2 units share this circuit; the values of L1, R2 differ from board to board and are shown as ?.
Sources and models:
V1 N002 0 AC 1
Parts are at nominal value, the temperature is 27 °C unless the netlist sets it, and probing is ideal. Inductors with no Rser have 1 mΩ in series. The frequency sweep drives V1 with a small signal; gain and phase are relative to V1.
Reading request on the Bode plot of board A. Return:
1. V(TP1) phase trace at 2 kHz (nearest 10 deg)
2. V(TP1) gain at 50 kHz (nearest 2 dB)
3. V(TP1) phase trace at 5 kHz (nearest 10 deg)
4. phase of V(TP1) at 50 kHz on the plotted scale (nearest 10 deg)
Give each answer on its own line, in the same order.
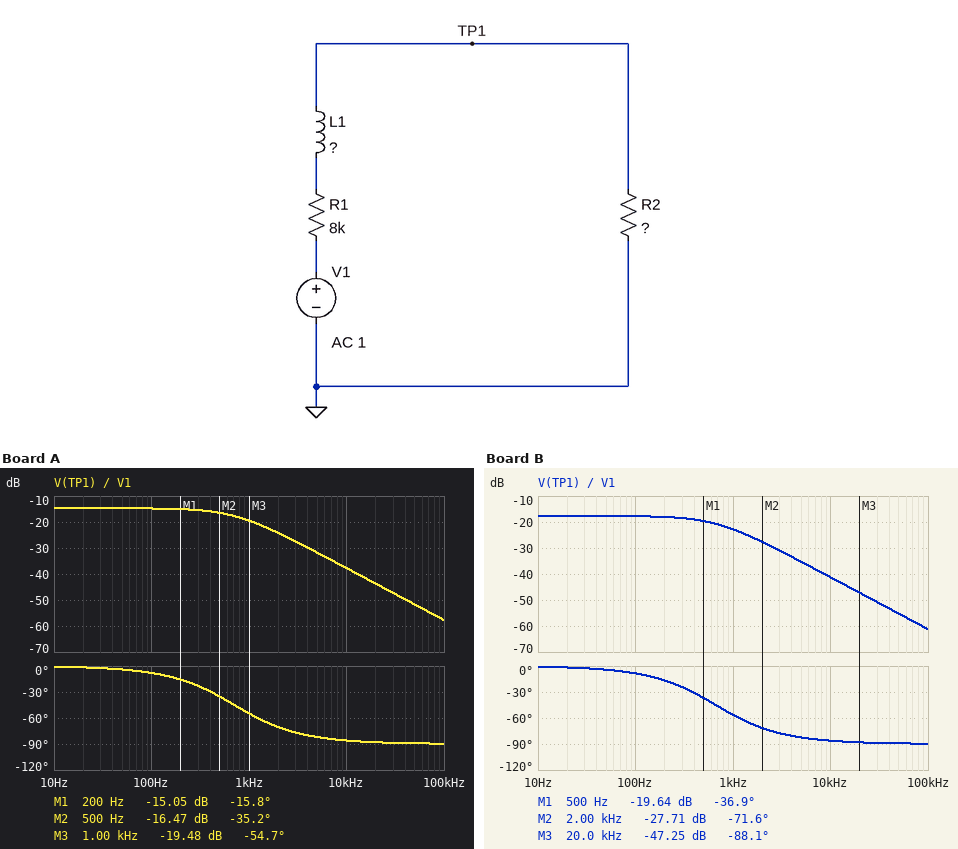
-70 deg
-52 dB
-80 deg
-90 deg
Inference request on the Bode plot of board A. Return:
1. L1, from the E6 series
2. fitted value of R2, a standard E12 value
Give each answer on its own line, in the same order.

2.2 H
1.8 kΩ
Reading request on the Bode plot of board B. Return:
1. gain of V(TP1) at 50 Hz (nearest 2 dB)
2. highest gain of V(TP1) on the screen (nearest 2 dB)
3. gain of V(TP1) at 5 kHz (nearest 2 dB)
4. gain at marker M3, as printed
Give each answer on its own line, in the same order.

-18 dB
-18 dB
-36 dB
-47.25 dB
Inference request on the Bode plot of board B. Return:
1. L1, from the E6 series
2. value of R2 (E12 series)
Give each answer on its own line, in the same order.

2.2 H
1.2 kΩ
